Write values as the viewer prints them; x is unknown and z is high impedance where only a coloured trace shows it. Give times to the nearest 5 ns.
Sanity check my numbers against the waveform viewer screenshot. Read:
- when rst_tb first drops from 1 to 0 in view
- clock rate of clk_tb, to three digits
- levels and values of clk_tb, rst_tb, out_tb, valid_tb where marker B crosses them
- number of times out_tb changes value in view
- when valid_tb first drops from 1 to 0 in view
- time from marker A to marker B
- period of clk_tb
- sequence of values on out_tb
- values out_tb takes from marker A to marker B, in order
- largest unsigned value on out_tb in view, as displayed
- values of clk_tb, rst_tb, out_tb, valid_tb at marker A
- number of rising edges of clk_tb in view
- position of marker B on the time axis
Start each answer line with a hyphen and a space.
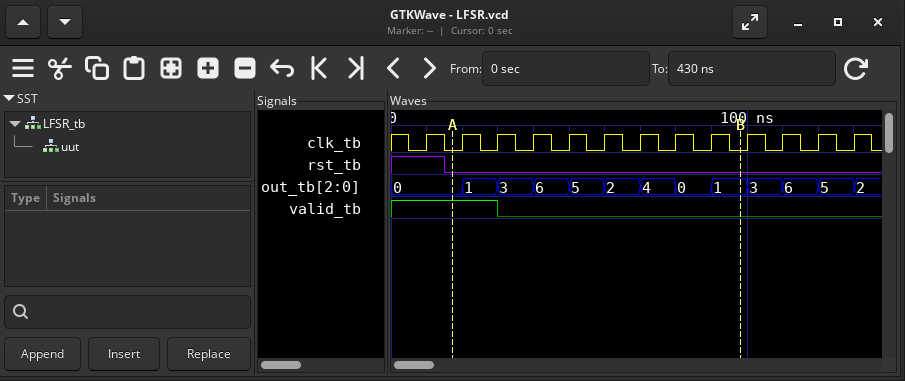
- 15 ns
- 100 MHz
- clk_tb=0, rst_tb=0, out_tb=1, valid_tb=0
- 12
- 30 ns
- 80 ns
- 10 ns
- 0, 1, 3, 6, 5, 2, 4, 0, 1, 3, 6, 5, 2
- 0, 1, 3, 6, 5, 2, 4, 0, 1
- 6
- clk_tb=0, rst_tb=0, out_tb=0, valid_tb=1
- 13
- 100 ns
